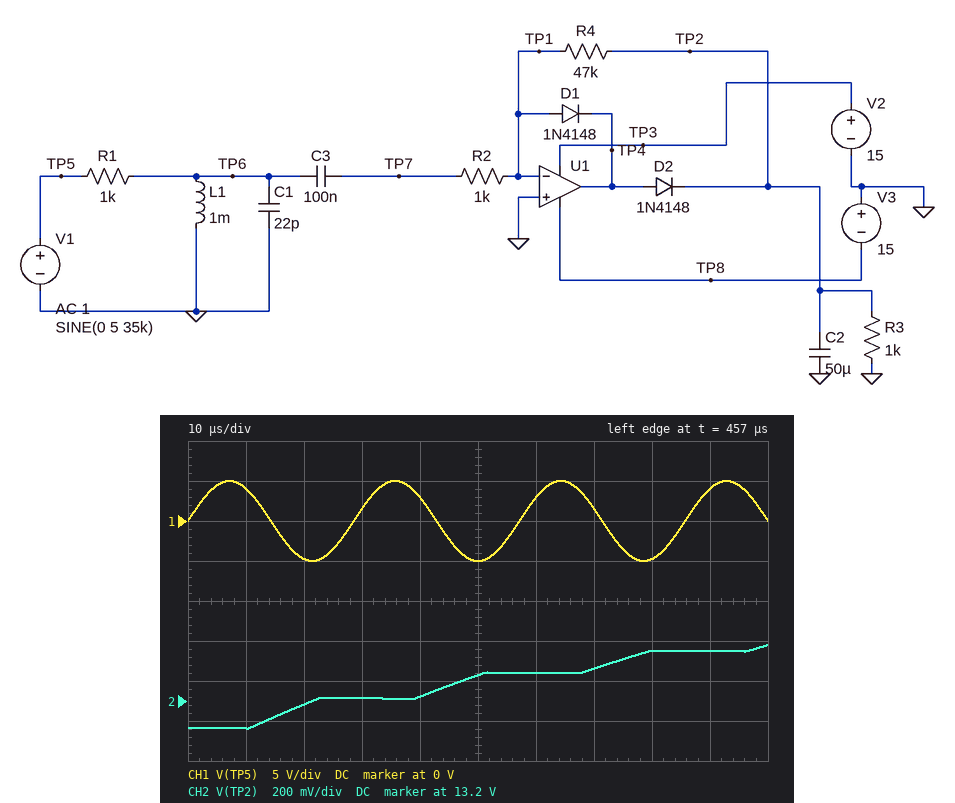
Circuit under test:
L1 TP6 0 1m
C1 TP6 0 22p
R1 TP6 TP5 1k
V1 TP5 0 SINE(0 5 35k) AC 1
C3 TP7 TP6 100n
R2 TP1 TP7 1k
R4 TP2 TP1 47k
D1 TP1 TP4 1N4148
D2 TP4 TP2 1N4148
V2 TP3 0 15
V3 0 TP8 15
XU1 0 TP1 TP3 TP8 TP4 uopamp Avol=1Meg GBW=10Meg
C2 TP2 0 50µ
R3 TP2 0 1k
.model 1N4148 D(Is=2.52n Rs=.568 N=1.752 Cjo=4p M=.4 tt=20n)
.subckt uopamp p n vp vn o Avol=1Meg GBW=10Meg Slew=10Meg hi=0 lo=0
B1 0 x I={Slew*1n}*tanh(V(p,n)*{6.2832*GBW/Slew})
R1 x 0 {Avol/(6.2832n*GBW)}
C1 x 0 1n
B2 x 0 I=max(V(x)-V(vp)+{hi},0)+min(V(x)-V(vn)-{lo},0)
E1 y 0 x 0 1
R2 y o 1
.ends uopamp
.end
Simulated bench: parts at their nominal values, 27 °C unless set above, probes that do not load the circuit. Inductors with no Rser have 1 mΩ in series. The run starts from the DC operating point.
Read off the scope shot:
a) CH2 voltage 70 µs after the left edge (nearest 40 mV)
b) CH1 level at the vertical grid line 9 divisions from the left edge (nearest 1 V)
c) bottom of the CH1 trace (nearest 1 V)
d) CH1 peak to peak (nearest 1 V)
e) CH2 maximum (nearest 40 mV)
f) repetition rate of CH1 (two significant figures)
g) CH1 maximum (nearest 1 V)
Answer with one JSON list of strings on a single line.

["13.36 V", "4 V", "-5 V", "10 V", "13.48 V", "35 kHz", "5 V"]
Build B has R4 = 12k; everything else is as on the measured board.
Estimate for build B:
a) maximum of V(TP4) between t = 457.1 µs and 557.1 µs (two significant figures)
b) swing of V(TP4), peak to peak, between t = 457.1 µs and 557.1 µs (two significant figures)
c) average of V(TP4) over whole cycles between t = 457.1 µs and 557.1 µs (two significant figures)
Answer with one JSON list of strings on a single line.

["13 V", "14 V", "1.5 V"]
